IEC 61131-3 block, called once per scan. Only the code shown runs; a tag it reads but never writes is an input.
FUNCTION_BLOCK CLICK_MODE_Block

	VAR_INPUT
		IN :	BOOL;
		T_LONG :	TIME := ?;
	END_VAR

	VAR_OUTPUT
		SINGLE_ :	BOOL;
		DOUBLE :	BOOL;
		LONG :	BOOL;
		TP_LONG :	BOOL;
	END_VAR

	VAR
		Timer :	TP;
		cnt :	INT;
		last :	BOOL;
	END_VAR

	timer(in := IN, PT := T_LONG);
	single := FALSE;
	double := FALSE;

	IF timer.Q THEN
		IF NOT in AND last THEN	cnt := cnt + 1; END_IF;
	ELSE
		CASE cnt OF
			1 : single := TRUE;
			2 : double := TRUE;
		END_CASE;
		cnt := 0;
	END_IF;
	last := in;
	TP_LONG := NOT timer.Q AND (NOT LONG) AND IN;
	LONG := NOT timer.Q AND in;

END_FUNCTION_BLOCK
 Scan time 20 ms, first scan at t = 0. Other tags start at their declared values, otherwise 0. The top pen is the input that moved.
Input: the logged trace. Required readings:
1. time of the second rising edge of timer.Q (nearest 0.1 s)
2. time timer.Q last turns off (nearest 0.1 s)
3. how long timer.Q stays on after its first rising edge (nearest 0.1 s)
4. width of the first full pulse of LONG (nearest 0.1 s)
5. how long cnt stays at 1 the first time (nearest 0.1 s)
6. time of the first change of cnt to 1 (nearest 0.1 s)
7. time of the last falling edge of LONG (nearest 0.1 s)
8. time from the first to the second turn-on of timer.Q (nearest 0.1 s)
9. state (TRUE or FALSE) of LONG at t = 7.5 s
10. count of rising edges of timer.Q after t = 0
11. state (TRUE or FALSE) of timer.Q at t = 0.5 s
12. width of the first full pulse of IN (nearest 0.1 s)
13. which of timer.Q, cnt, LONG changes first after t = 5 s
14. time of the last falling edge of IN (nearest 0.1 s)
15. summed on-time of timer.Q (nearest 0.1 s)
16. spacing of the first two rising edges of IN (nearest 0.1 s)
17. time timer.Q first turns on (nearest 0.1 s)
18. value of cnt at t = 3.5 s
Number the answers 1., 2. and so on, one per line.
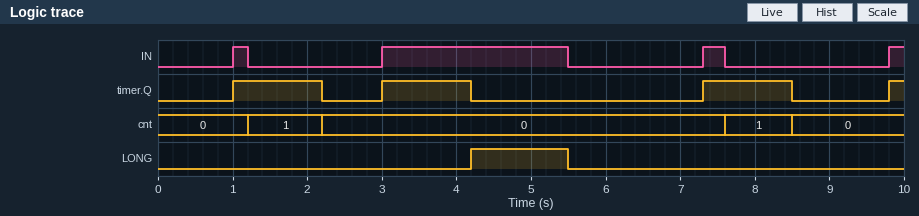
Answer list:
1. 3.0 s
2. 8.5 s
3. 1.2 s
4. 1.3 s
5. 1.0 s
6. 1.2 s
7. 5.5 s
8. 2.0 s
9. FALSE
10. 4
11. FALSE
12. 0.2 s
13. LONG
14. 7.6 s
15. 3.8 s
16. 2.0 s
17. 1.0 s
18. 0
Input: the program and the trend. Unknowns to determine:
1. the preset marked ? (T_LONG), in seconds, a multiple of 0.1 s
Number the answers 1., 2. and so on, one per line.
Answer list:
1. 1.2 s
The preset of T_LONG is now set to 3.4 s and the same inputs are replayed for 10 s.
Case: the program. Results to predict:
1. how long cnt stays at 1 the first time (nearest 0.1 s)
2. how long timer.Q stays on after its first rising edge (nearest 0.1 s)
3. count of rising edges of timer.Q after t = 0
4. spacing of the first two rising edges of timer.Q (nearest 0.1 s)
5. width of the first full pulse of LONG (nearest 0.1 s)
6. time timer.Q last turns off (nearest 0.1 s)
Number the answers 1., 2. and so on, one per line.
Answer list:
1. 3.2 s
2. 3.4 s
3. 2
4. 6.3 s
5. 1.1 s
6. 4.4 s
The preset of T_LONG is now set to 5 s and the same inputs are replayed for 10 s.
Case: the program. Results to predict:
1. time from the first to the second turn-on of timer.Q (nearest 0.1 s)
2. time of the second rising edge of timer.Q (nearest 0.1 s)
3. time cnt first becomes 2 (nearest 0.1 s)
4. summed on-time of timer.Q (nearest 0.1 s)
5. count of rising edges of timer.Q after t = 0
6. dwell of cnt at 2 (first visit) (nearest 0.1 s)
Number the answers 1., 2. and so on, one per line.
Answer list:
1. 6.3 s
2. 7.3 s
3. 5.5 s
4. 7.7 s
5. 2
6. 0.5 s
